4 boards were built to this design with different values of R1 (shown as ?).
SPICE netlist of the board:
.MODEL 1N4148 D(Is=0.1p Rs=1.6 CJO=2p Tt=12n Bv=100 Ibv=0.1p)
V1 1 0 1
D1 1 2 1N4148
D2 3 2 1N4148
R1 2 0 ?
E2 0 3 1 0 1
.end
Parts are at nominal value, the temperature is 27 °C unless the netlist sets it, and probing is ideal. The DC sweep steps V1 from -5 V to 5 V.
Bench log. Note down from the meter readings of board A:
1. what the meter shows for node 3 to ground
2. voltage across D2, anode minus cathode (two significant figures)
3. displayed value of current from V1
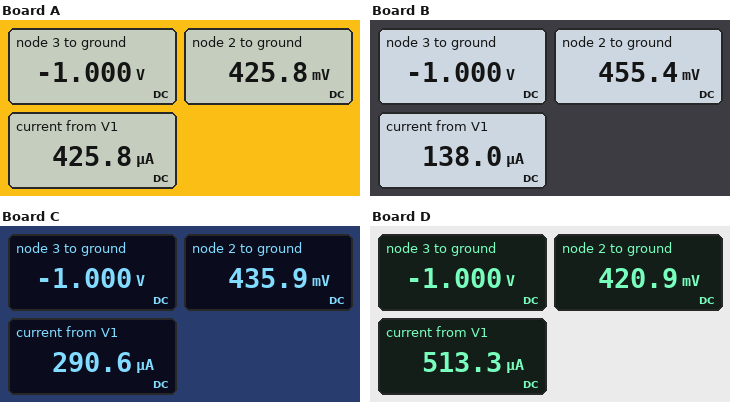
-1.000 V
-1.4 V
425.8 µA
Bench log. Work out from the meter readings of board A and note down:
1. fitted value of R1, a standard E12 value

1 kΩ
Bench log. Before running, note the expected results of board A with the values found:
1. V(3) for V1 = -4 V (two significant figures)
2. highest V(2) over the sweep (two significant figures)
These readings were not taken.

4.0 V
4.4 V
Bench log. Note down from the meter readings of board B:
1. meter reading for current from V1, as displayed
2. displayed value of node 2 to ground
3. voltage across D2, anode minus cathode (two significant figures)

138.0 µA
455.4 mV
-1.5 V
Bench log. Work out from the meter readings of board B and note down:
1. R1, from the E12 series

3.3 kΩ
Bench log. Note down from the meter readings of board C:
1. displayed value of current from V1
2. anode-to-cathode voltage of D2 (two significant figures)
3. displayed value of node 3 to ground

290.6 µA
-1.4 V
-1.000 V
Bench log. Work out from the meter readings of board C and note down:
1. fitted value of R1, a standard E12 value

1.5 kΩ
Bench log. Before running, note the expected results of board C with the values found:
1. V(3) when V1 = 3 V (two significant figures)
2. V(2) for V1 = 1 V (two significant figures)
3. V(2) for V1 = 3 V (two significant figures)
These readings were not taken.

-3.0 V
440 mV
2.4 V
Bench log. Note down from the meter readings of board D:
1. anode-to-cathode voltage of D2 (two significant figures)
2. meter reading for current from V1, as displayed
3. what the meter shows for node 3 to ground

-1.4 V
513.3 µA
-1.000 V
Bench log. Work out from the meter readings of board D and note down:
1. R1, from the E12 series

820 Ω
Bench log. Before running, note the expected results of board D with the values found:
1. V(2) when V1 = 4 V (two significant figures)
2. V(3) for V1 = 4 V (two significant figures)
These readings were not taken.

3.4 V
-4.0 V
